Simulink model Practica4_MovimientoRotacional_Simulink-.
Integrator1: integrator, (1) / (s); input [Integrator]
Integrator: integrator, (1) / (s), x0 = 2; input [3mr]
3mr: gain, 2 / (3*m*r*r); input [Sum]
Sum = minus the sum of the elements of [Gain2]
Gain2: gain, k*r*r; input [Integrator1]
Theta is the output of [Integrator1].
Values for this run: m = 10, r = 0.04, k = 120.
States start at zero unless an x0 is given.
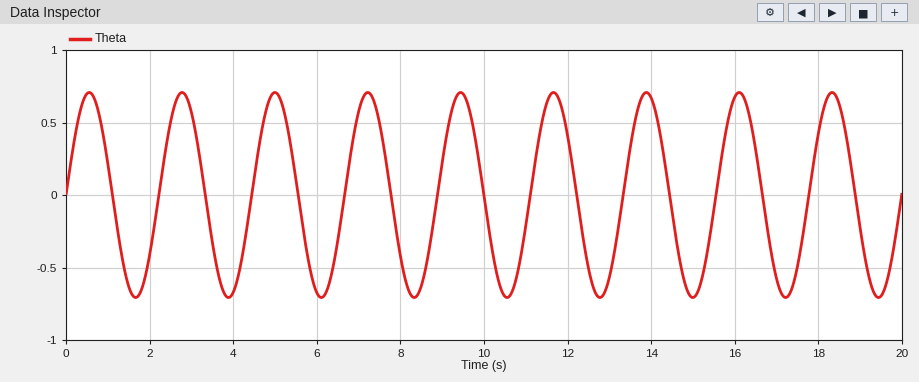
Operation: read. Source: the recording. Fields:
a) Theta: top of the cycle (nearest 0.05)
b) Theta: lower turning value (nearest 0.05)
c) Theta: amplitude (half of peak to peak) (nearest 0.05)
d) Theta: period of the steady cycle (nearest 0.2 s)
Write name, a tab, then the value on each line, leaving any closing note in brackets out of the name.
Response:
Theta: top of the cycle	0.70
Theta: lower turning value	-0.70
Theta: amplitude (half of peak to peak)	0.70
Theta: period of the steady cycle	2.2 s
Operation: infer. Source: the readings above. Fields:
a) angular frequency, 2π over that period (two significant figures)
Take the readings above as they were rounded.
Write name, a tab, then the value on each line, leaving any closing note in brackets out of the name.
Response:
angular frequency, 2π over that period	2.9 rad/s
